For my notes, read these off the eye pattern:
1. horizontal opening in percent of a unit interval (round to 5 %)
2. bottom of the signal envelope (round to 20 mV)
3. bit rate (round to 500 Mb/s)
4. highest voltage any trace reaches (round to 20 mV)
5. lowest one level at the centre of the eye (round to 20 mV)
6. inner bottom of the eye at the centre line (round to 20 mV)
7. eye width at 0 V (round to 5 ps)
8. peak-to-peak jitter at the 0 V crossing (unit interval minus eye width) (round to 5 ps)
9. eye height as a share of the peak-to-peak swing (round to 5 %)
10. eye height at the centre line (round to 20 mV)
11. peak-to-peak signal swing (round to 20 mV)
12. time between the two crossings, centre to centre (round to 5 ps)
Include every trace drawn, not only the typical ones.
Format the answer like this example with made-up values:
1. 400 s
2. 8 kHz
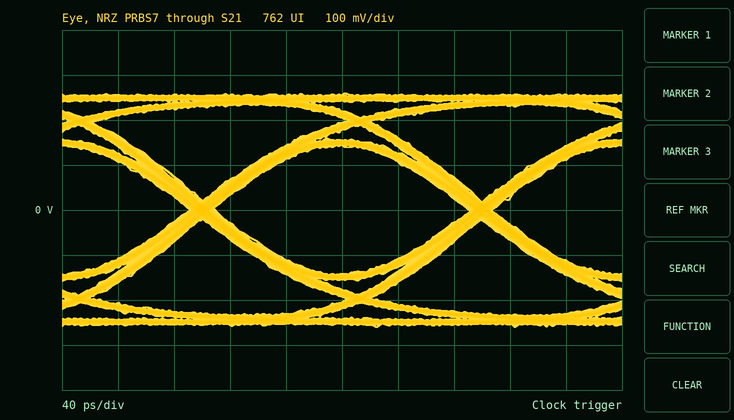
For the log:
1. 90 %
2. -260 mV
3. 5.0 Gb/s
4. 260 mV
5. 140 mV
6. -140 mV
7. 180 ps
8. 20 ps
9. 55 %
10. 280 mV
11. 520 mV
12. 200 ps
